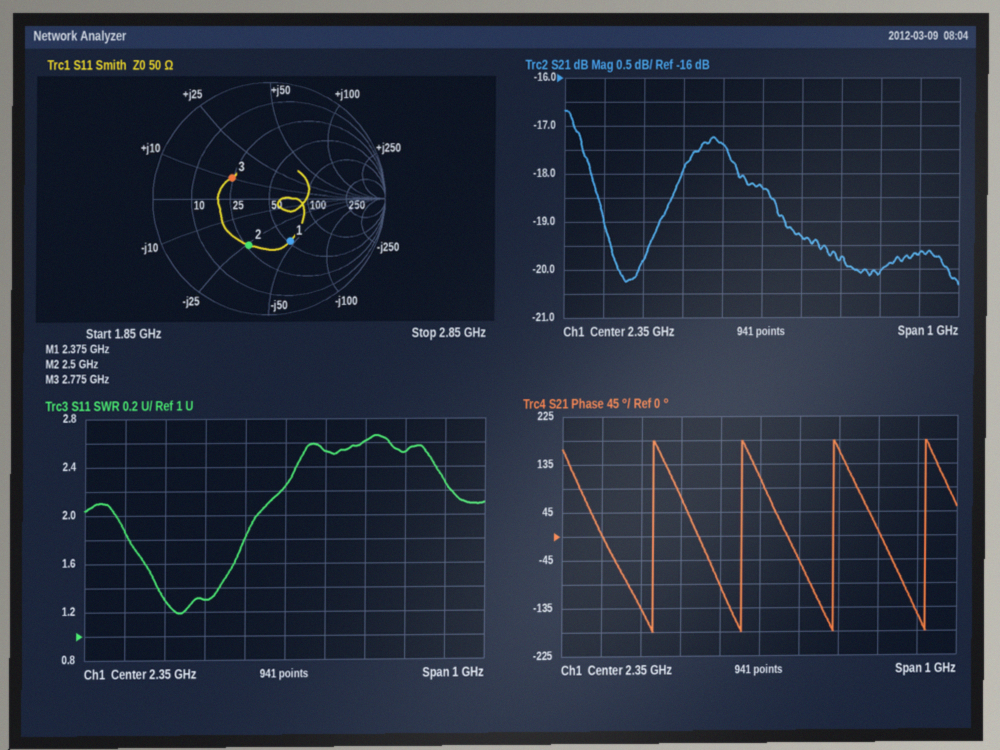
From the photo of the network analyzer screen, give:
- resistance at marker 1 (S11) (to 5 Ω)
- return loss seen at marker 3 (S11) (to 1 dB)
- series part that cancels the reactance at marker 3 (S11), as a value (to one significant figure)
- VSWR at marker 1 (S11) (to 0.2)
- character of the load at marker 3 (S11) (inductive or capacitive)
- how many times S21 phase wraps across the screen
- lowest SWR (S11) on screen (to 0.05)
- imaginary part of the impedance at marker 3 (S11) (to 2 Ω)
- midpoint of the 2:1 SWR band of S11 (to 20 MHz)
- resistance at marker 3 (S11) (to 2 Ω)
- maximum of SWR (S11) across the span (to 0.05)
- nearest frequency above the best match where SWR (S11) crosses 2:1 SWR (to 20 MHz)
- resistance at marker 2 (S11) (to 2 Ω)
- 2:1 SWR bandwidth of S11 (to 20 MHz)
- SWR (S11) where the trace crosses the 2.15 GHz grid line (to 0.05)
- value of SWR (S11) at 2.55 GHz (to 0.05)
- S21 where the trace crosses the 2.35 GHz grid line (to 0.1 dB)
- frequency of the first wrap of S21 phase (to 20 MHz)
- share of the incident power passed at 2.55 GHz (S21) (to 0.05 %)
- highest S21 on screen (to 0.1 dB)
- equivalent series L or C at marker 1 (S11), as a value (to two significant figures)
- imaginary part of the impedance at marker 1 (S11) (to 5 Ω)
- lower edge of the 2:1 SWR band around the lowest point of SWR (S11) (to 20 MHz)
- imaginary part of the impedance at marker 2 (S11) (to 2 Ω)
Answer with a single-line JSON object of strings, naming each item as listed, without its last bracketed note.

{"resistance at marker 1 (S11)": "50 Ω", "return loss seen at marker 3 (S11)": "9 dB", "series part that cancels the reactance at marker 3 (S11), as a value": "6 pF", "VSWR at marker 1 (S11)": "2.4", "character of the load at marker 3 (S11)": "inductive", "how many times S21 phase wraps across the screen": "4", "lowest SWR (S11) on screen": "1.20", "imaginary part of the impedance at marker 3 (S11)": "+10 Ω", "midpoint of the 2:1 SWR band of S11": "2.10 GHz", "resistance at marker 3 (S11)": "24 Ω", "maximum of SWR (S11) across the span": "2.65", "nearest frequency above the best match where SWR (S11) crosses 2:1 SWR": "2.28 GHz", "resistance at marker 2 (S11)": "26 Ω", "2:1 SWR bandwidth of S11": "360 MHz", "SWR (S11) where the trace crosses the 2.15 GHz grid line": "1.30", "value of SWR (S11) at 2.55 GHz": "2.60", "S21 where the trace crosses the 2.35 GHz grid line": "-18.3 dB", "frequency of the first wrap of S21 phase": "2.08 GHz", "share of the incident power passed at 2.55 GHz (S21)": "1.05 %", "highest S21 on screen": "-16.7 dB", "equivalent series L or C at marker 1 (S11), as a value": "1.5 pF", "imaginary part of the impedance at marker 1 (S11)": "-45 Ω", "lower edge of the 2:1 SWR band around the lowest point of SWR (S11)": "1.92 GHz", "imaginary part of the impedance at marker 2 (S11)": "-26 Ω"}
